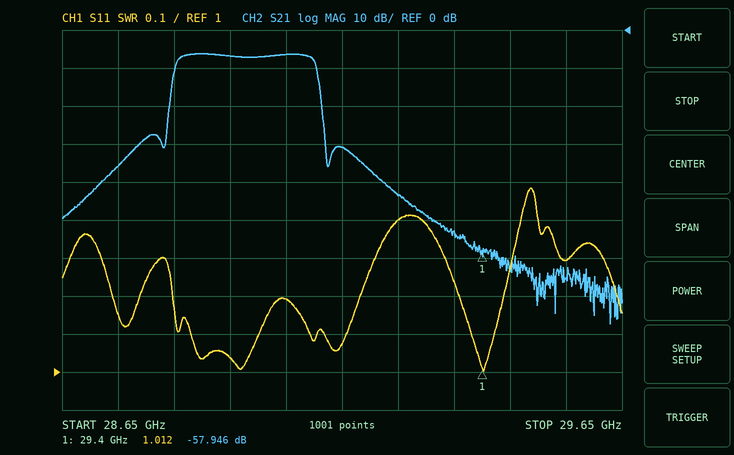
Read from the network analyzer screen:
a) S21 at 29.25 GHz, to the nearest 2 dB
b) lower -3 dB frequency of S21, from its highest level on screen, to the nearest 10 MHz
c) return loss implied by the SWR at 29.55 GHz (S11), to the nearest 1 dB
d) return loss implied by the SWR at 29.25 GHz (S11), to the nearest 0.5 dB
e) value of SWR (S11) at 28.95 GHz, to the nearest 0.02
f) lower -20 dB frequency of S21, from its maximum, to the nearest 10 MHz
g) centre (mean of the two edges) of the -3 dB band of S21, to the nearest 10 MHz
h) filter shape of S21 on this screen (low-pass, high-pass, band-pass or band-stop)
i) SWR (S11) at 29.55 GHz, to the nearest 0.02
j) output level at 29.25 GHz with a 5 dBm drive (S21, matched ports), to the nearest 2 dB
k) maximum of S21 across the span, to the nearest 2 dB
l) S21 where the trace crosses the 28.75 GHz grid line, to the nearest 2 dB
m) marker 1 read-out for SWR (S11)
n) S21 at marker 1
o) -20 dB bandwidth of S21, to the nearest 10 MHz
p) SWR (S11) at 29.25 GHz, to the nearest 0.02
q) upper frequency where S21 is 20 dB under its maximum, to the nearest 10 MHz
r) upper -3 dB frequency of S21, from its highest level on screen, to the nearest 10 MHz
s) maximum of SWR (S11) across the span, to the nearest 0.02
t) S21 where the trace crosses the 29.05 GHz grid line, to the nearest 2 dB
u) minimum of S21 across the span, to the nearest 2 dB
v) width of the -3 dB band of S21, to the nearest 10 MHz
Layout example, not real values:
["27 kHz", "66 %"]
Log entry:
["-44 dB", "28.85 GHz", "18 dB", "15.5 dB", "1.04", "28.84 GHz", "28.98 GHz", "band-pass", "1.30", "-38 dBm", "-6 dB", "-36 dB", "1.012", "-57.946 dB", "280 MHz", "1.40", "29.12 GHz", "29.10 GHz", "1.48", "-6 dB", "-78 dB", "250 MHz"]
